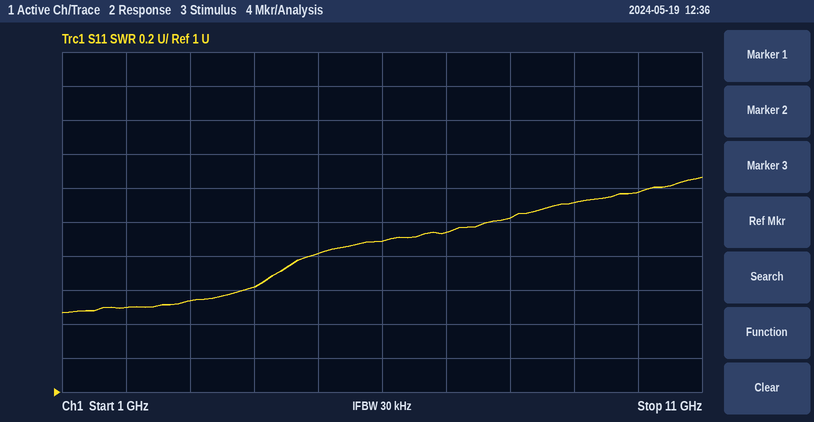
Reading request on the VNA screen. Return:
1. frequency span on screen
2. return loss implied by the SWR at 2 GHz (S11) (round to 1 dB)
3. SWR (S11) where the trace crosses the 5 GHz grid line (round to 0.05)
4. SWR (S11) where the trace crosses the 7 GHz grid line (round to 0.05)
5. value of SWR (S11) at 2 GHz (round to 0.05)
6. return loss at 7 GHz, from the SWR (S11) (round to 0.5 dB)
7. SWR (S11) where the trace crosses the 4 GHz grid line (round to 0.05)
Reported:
10 GHz
14 dB
1.80
1.95
1.50
10.0 dB
1.60
